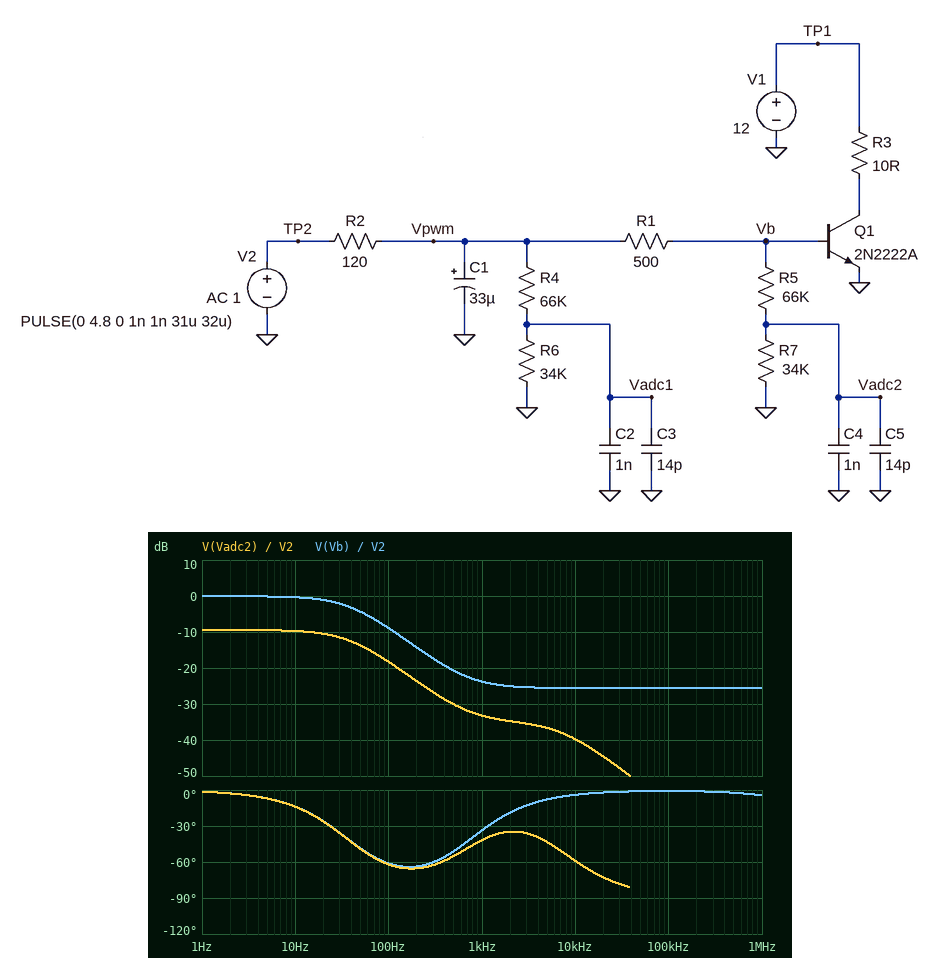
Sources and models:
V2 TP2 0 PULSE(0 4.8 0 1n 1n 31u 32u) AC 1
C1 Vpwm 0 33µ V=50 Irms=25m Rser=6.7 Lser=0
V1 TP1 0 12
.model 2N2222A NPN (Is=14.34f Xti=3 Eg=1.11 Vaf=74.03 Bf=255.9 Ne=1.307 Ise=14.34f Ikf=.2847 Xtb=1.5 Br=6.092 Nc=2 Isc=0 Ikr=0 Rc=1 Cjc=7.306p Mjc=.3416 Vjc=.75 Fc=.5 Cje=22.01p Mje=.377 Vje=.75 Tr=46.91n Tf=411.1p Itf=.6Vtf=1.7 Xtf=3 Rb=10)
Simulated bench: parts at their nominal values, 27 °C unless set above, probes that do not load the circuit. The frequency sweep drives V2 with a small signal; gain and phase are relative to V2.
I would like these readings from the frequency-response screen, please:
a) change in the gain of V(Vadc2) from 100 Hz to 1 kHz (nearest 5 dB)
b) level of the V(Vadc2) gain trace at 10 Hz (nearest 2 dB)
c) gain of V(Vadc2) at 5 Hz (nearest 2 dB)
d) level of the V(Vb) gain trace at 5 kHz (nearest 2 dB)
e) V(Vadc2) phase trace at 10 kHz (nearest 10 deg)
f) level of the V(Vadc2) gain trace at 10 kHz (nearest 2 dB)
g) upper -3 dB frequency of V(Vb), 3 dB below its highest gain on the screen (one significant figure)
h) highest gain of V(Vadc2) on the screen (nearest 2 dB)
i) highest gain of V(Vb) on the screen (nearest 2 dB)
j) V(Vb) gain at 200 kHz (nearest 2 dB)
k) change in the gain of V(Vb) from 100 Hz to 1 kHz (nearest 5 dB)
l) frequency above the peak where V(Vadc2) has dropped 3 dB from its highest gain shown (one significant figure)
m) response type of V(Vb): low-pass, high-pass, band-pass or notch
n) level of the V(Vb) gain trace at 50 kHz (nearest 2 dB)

-15 dB
-10 dB
-10 dB
-26 dB
-60 deg
-40 dB
40 Hz
-10 dB
0 dB
-26 dB
-15 dB
40 Hz
low-pass
-26 dB
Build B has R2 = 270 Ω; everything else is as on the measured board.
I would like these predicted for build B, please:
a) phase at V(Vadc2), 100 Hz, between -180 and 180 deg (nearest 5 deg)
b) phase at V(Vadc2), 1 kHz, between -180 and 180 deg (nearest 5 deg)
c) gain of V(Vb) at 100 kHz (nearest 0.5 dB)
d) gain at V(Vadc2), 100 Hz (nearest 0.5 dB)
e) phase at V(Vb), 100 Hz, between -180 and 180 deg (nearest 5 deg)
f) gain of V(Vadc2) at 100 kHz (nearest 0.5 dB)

-75 deg
-45 deg
-32.5 dB
-24.5 dB
-70 deg
-65.0 dB
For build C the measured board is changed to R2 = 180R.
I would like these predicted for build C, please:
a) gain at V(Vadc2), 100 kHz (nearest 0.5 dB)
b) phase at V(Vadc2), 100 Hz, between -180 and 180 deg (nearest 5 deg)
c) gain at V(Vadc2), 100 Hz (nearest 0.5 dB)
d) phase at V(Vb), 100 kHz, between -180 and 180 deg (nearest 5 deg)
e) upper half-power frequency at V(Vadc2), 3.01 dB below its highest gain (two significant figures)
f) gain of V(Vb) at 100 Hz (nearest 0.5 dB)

-61.5 dB
-70 deg
-21.5 dB
0 deg
26 Hz
-12.0 dB
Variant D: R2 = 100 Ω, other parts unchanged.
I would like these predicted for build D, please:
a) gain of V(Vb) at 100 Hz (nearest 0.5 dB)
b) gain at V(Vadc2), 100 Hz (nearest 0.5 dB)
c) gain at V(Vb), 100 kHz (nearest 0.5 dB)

-7.5 dB
-17.0 dB
-24.0 dB
